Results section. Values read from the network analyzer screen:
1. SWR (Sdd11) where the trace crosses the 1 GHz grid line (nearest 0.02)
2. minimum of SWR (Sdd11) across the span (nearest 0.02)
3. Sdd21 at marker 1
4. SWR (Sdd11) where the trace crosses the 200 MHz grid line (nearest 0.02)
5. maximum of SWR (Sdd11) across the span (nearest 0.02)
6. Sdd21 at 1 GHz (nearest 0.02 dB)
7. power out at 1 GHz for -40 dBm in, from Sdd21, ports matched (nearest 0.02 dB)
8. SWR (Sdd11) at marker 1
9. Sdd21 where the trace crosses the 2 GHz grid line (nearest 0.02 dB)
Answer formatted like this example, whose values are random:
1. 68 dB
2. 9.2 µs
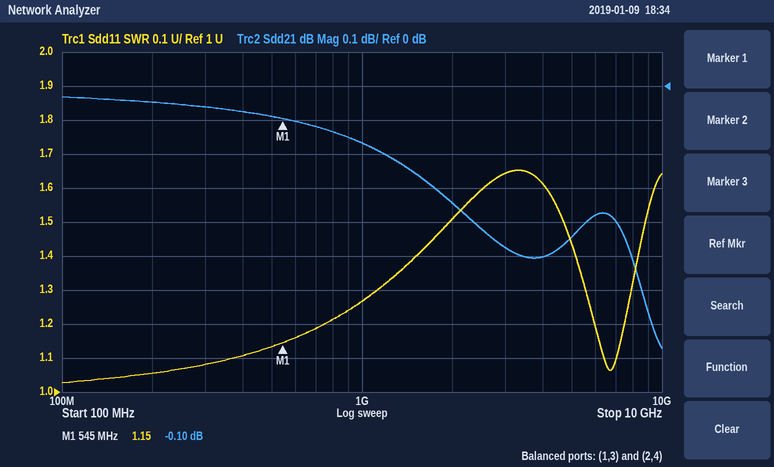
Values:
1. 1.26
2. 1.02
3. -0.10 dB
4. 1.06
5. 1.66
6. -0.16 dB
7. -40.16 dBm
8. 1.15
9. -0.34 dB
